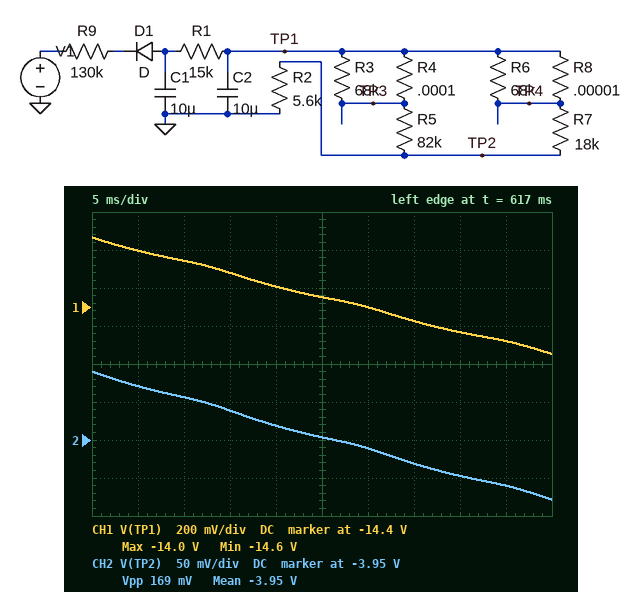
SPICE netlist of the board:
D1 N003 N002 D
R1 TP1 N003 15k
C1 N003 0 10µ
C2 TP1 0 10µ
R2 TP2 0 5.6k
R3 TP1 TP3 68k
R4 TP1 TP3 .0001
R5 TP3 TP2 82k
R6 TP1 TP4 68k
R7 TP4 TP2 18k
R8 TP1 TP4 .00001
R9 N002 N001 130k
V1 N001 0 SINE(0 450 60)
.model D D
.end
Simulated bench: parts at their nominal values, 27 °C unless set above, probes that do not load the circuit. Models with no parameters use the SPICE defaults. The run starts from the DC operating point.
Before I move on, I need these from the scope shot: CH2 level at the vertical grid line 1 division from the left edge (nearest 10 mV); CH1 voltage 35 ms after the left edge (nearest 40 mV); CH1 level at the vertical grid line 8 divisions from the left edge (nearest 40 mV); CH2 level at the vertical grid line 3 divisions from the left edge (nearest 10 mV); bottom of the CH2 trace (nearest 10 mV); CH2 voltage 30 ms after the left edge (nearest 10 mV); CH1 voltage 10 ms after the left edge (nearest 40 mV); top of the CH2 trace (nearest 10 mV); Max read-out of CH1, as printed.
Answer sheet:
-3.88 V
-14.48 V
-14.52 V
-3.91 V
-4.03 V
-3.96 V
-14.16 V
-3.86 V
-14.0 V
